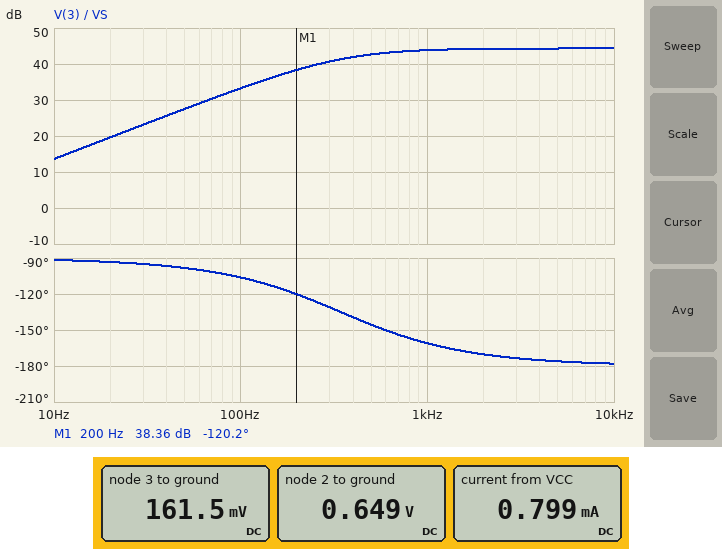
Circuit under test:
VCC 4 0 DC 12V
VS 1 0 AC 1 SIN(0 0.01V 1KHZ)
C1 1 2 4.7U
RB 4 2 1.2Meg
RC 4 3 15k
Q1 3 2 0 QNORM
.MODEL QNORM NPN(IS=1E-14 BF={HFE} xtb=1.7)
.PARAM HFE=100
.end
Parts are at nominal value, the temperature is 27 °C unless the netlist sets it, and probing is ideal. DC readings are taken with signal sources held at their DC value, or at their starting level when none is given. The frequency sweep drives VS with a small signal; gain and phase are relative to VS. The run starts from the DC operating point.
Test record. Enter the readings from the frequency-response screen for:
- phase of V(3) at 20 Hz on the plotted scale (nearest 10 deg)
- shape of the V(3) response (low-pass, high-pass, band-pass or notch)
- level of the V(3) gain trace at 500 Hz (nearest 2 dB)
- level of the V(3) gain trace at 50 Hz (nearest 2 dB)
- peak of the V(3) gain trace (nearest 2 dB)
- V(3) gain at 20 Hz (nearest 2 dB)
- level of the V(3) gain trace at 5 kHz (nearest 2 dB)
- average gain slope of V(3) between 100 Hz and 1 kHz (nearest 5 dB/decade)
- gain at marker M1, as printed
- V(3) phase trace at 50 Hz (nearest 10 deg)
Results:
-90 deg
high-pass
42 dB
28 dB
44 dB
20 dB
44 dB
10 dB/decade
38.36 dB
-100 deg
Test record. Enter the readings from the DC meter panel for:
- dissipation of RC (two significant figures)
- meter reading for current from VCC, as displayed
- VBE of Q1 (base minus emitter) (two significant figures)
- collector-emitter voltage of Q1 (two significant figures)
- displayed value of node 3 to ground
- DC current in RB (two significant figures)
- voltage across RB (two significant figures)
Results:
9.3 mW
0.799 mA
650 mV
160 mV
161.5 mV
9.5 µA
11 V
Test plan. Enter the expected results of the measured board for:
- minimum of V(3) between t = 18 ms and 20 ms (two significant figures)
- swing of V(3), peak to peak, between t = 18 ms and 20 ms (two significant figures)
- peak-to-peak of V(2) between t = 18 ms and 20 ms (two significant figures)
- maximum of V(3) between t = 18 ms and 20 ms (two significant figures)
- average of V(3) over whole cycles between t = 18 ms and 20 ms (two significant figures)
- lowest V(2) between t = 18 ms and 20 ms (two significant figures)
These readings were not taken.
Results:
89 mV
6.0 V
20 mV
6.1 V
3.1 V
630 mV
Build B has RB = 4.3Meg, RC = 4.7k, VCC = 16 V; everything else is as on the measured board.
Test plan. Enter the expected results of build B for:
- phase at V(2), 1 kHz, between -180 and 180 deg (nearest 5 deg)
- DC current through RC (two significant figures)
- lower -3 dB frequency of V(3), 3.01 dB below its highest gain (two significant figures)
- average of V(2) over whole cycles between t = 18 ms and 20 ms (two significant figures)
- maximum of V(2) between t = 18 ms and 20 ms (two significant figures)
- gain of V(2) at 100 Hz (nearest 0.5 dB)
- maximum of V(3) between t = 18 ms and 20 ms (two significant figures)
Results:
0 deg
360 µA
4.7 Hz
630 mV
640 mV
0 dB
15 V
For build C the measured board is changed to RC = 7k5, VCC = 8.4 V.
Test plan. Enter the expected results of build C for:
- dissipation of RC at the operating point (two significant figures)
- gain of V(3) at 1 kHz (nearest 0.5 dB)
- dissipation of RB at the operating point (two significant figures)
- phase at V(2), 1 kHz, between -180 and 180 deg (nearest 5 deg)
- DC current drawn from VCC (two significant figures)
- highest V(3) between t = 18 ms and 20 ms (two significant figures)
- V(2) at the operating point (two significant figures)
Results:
3.1 mW
45.5 dB
50 µW
0 deg
650 µA
5.2 V
640 mV
